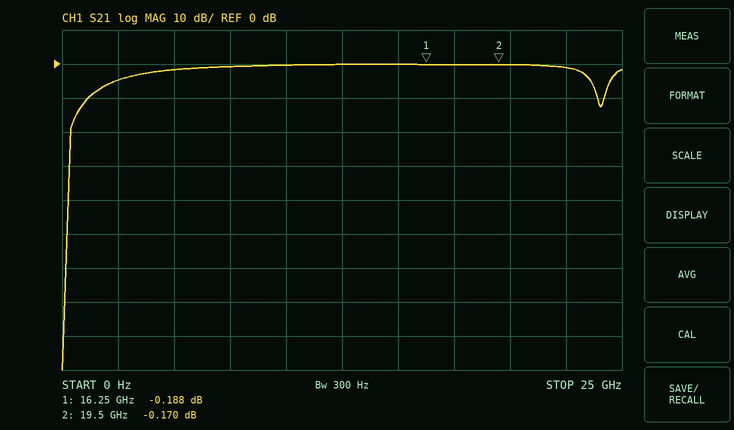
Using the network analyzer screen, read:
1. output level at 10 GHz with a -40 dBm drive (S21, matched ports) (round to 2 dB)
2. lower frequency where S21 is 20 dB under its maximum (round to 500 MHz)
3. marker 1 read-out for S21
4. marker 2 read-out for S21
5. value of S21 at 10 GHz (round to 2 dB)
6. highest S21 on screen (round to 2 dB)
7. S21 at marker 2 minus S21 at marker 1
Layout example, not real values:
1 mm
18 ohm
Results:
-40 dBm
500 MHz
-0.188 dB
-0.170 dB
0 dB
0 dB
0.018 dB
